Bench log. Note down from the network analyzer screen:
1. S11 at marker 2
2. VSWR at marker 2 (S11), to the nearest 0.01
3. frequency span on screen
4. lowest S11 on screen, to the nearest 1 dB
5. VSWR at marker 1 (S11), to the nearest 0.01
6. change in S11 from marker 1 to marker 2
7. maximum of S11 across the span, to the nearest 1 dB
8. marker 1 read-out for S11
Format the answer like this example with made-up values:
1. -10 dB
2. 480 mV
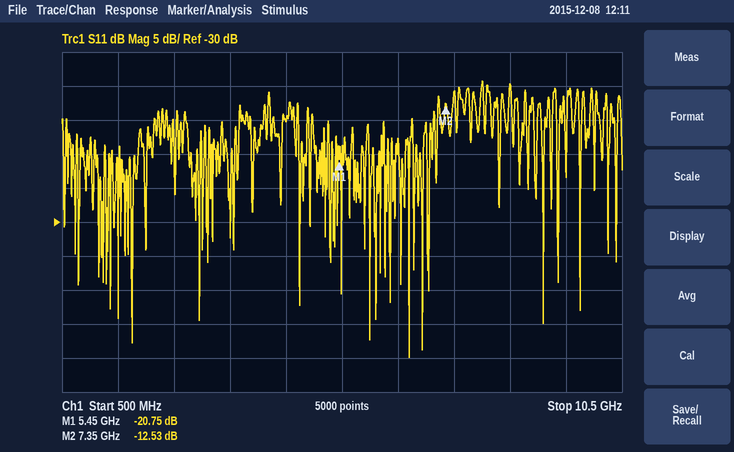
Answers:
1. -12.53 dB
2. 1.62
3. 10 GHz
4. -50 dB
5. 1.20
6. 8.22 dB
7. -9 dB
8. -20.75 dB
